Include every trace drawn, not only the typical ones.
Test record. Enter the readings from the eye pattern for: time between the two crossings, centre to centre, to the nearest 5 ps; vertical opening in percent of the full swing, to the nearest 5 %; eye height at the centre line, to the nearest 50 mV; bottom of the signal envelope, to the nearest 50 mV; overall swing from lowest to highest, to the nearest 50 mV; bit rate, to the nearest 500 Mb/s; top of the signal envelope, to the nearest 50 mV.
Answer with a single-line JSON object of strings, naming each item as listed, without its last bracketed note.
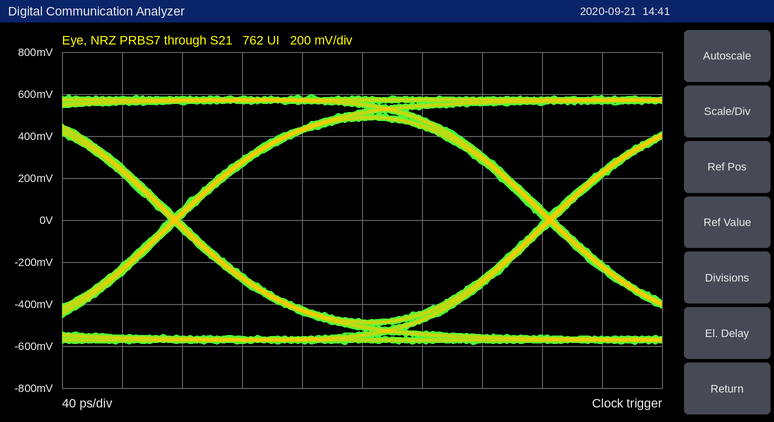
{"time between the two crossings, centre to centre, to the nearest 5 ps": "250 ps", "vertical opening in percent of the full swing, to the nearest 5 %": "80 %", "eye height at the centre line, to the nearest 50 mV": "950 mV", "bottom of the signal envelope, to the nearest 50 mV": "-600 mV", "overall swing from lowest to highest, to the nearest 50 mV": "1.20 V", "bit rate, to the nearest 500 Mb/s": "4.0 Gb/s", "top of the signal envelope, to the nearest 50 mV": "600 mV"}
